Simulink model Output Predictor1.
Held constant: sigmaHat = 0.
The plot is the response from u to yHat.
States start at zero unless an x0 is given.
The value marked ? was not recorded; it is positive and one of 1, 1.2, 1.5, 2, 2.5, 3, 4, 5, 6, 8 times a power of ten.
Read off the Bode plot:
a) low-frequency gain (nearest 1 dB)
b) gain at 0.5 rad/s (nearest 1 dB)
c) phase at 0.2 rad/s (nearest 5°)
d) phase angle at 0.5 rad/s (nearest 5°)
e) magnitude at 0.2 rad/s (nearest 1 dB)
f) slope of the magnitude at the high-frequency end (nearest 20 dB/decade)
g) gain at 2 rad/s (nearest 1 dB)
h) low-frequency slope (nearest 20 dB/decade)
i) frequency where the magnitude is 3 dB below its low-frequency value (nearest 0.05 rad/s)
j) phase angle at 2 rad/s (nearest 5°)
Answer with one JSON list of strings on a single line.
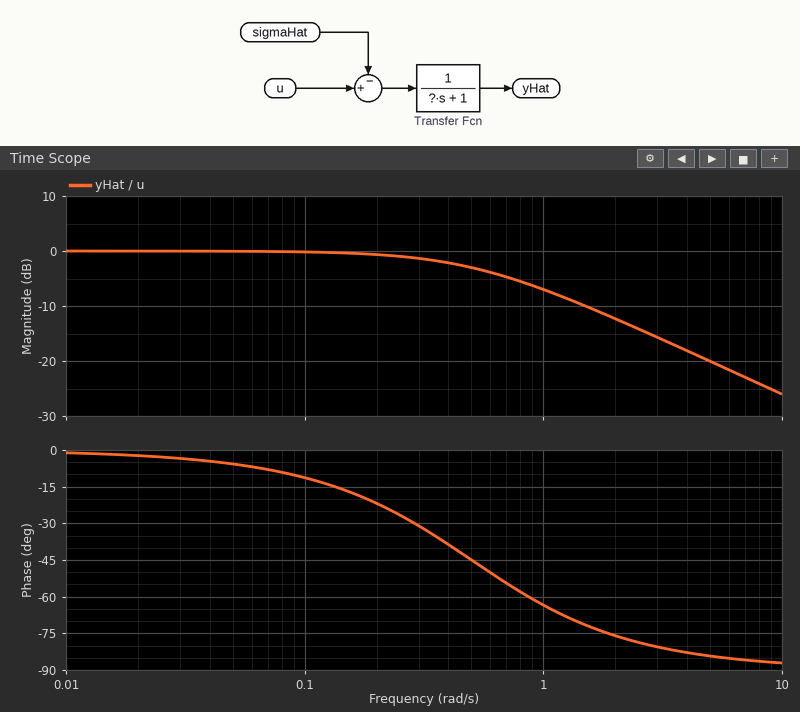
["0 dB", "-3 dB", "-20°", "-45°", "-1 dB", "-20 dB/decade", "-12 dB", "0 dB/decade", "0.50 rad/s", "-75°"]
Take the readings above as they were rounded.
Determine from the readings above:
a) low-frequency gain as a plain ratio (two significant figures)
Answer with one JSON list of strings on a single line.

["1.0"]
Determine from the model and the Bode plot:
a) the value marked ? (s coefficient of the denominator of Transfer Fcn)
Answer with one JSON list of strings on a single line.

["2"]
